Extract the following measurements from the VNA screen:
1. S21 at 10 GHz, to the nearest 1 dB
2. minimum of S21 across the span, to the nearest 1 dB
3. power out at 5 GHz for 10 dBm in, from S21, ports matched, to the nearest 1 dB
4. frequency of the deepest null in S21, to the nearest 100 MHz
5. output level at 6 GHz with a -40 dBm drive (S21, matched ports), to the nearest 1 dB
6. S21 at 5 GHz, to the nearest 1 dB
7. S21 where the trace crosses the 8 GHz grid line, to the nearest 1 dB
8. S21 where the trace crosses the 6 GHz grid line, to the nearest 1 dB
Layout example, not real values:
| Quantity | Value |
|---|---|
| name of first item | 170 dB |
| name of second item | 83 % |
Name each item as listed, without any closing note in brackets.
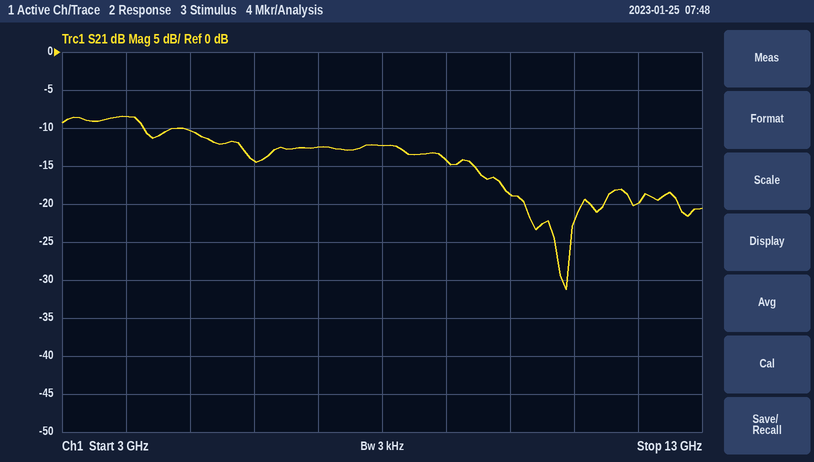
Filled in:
| Quantity | Value |
|---|---|
| S21 at 10 GHz, to the nearest 1 dB | -19 dB |
| minimum of S21 across the span, to the nearest 1 dB | -31 dB |
| power out at 5 GHz for 10 dBm in, from S21, ports matched, to the nearest 1 dB | 0 dBm |
| frequency of the deepest null in S21, to the nearest 100 MHz | 10.9 GHz |
| output level at 6 GHz with a -40 dBm drive (S21, matched ports), to the nearest 1 dB | -54 dBm |
| S21 at 5 GHz, to the nearest 1 dB | -10 dB |
| S21 where the trace crosses the 8 GHz grid line, to the nearest 1 dB | -12 dB |
| S21 where the trace crosses the 6 GHz grid line, to the nearest 1 dB | -14 dB |
